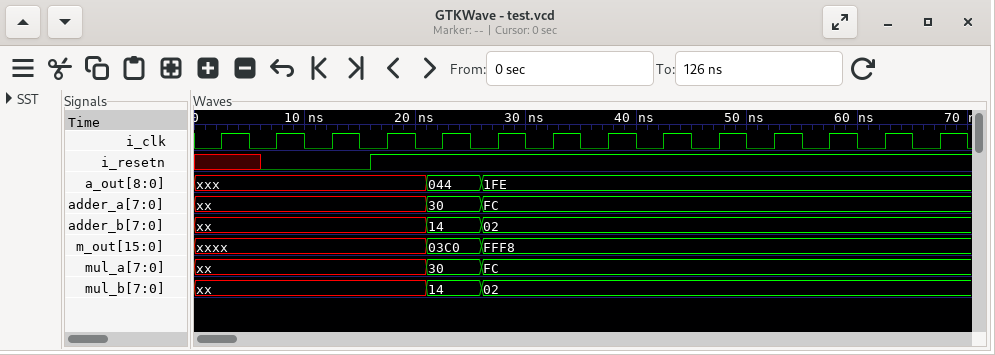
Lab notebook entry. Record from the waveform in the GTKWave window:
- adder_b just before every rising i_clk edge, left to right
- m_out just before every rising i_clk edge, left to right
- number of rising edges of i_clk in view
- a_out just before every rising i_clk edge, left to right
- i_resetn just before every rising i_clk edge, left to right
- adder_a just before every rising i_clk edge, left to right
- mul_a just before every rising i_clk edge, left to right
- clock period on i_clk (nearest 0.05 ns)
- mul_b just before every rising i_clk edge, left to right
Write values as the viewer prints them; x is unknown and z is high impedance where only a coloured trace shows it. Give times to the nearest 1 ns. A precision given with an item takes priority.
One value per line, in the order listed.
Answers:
xx, xx, xx, xx, 14, 02, 02, 02, 02, 02, 02, 02, 02, 02
xxxx, xxxx, xxxx, xxxx, 03C0, FFF8, FFF8, FFF8, FFF8, FFF8, FFF8, FFF8, FFF8, FFF8
14
xxx, xxx, xxx, xxx, 044, 1FE, 1FE, 1FE, 1FE, 1FE, 1FE, 1FE, 1FE, 1FE
x 0 0 1 1 1 1 1 1 1 1 1 1 1
xx, xx, xx, xx, 30, FC, FC, FC, FC, FC, FC, FC, FC, FC
xx, xx, xx, xx, 30, FC, FC, FC, FC, FC, FC, FC, FC, FC
5 ns
xx, xx, xx, xx, 14, 02, 02, 02, 02, 02, 02, 02, 02, 02
